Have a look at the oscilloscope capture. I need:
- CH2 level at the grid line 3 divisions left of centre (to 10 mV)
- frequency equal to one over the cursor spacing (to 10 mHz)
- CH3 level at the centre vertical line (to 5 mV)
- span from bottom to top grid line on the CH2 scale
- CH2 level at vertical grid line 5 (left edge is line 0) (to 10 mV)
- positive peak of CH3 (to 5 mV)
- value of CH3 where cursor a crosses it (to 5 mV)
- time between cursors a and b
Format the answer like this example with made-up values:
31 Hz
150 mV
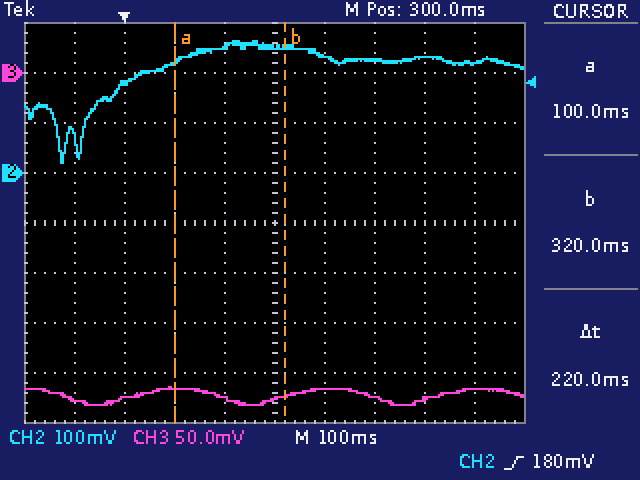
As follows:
180 mV
4.55 Hz
-325 mV
800 mV
250 mV
-315 mV
-315 mV
220 ms
